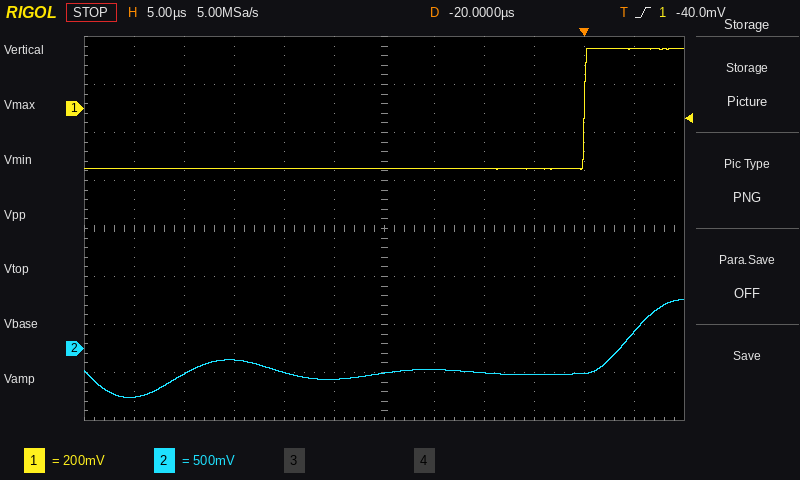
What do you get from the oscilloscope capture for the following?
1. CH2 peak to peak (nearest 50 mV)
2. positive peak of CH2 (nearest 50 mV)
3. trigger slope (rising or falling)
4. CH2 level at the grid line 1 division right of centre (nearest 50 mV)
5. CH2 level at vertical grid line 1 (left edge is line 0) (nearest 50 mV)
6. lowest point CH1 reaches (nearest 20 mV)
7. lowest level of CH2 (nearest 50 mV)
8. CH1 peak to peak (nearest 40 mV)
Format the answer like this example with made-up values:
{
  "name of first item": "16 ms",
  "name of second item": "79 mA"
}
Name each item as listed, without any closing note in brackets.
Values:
{
  "CH2 peak to peak": "1.00 V",
  "positive peak of CH2": "500 mV",
  "trigger slope": "rising",
  "CH2 level at the grid line 1 division right of centre": "-200 mV",
  "CH2 level at vertical grid line 1 (left edge is line 0)": "-500 mV",
  "lowest point CH1 reaches": "-260 mV",
  "lowest level of CH2": "-500 mV",
  "CH1 peak to peak": "520 mV"
}
